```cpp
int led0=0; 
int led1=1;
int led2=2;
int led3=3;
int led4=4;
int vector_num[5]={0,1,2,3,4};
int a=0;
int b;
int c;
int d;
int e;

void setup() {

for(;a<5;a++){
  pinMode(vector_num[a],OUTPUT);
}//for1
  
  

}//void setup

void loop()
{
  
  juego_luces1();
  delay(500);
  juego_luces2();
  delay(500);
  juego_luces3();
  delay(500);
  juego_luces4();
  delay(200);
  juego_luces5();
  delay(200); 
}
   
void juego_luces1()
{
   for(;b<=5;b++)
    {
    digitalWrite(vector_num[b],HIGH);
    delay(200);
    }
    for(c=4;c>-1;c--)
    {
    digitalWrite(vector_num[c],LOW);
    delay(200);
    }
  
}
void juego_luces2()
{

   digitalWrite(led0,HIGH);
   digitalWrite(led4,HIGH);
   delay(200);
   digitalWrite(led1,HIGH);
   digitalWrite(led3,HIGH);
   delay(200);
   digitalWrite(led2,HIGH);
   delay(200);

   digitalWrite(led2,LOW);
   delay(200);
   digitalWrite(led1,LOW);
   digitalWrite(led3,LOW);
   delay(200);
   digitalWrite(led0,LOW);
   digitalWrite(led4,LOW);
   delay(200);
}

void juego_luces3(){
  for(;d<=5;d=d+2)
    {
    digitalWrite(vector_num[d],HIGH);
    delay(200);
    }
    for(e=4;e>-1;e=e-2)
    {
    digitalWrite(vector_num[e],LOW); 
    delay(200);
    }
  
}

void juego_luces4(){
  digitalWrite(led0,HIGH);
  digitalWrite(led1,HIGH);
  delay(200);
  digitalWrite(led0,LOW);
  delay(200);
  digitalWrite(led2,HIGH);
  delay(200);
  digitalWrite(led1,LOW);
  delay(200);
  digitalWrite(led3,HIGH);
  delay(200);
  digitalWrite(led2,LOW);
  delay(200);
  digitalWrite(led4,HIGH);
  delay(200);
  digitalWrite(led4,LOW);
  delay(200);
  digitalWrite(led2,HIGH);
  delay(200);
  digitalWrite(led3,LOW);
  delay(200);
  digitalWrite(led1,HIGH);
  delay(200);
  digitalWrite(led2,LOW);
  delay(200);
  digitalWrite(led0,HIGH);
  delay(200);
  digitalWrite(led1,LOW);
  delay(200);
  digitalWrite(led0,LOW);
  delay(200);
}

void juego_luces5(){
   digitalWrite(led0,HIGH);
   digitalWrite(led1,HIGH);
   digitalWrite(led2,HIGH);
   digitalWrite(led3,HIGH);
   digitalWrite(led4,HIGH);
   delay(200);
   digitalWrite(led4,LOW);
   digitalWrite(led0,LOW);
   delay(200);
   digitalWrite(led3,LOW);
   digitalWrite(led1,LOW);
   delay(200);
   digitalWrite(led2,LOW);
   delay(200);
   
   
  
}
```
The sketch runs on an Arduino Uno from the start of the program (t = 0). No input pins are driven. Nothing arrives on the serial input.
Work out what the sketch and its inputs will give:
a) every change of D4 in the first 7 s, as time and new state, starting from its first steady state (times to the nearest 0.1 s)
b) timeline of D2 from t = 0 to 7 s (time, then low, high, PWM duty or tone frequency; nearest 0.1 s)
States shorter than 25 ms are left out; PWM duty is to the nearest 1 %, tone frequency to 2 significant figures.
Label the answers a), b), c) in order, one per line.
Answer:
a) 0 s low; 0.8 s high; 1.2 s low; 2.7 s high; 3.7 s low; 4.8 s high; 5 s low
b) 0 s low; 0.4 s high; 1.6 s low; 3.1 s high; 3.3 s low; 4.6 s high; 5.2 s low; 6.5 s high
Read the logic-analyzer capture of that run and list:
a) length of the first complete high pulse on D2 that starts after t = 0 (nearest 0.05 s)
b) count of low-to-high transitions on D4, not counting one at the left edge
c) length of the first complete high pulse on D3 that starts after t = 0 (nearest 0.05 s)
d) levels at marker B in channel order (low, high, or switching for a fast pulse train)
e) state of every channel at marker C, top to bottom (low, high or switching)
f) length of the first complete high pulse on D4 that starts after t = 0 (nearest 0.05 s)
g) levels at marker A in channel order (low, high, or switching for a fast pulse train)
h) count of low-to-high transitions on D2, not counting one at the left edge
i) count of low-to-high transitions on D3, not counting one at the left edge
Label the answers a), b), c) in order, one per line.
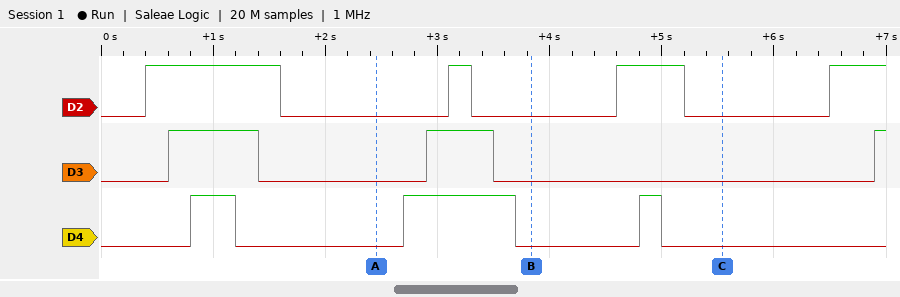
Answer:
a) 1.20 s
b) 3
c) 0.80 s
d) D2 low, D3 low, D4 low
e) D2 low, D3 low, D4 low
f) 0.40 s
g) D2 low, D3 low, D4 low
h) 4
i) 3
